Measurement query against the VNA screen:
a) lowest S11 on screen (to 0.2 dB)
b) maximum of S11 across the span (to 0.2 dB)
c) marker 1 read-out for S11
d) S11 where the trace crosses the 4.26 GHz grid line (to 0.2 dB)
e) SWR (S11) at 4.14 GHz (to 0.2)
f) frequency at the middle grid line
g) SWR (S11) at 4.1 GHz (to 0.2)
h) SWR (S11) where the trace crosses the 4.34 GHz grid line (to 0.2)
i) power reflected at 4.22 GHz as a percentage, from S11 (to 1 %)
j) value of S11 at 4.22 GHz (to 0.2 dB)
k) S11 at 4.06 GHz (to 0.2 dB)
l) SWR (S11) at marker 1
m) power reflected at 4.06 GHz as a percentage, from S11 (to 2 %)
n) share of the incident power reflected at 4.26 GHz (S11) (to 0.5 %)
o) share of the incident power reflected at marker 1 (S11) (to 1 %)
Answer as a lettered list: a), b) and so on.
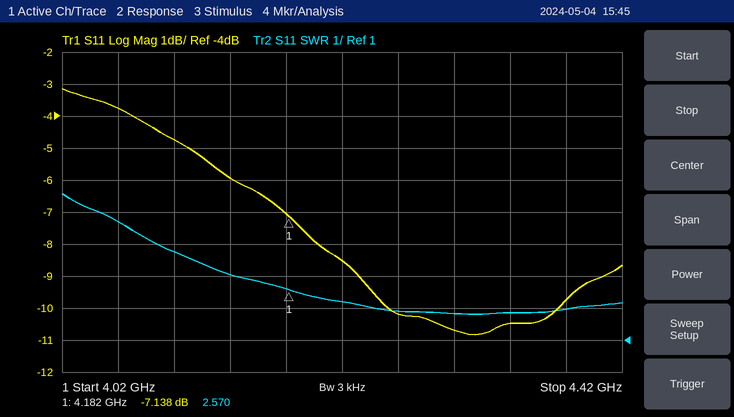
a) -10.8 dB
b) -3.2 dB
c) -7.138 dB
d) -10.2 dB
e) 3.0
f) 4.22 GHz
g) 3.8
h) 1.8
i) 14 %
j) -8.6 dB
k) -3.8 dB
l) 2.570
m) 42 %
n) 9.5 %
o) 19 %
